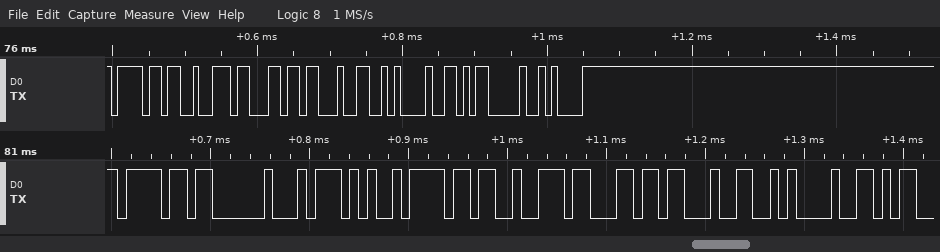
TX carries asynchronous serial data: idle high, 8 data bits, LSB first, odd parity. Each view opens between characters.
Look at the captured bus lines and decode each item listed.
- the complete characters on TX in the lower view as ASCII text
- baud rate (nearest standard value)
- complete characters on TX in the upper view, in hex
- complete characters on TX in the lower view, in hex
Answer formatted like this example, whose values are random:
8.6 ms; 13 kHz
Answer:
"o World!"; 115200 baud; 6F, 72, 6C, 64, 21, 0D, 0A; 6F, 20, 57, 6F, 72, 6C, 64, 21
